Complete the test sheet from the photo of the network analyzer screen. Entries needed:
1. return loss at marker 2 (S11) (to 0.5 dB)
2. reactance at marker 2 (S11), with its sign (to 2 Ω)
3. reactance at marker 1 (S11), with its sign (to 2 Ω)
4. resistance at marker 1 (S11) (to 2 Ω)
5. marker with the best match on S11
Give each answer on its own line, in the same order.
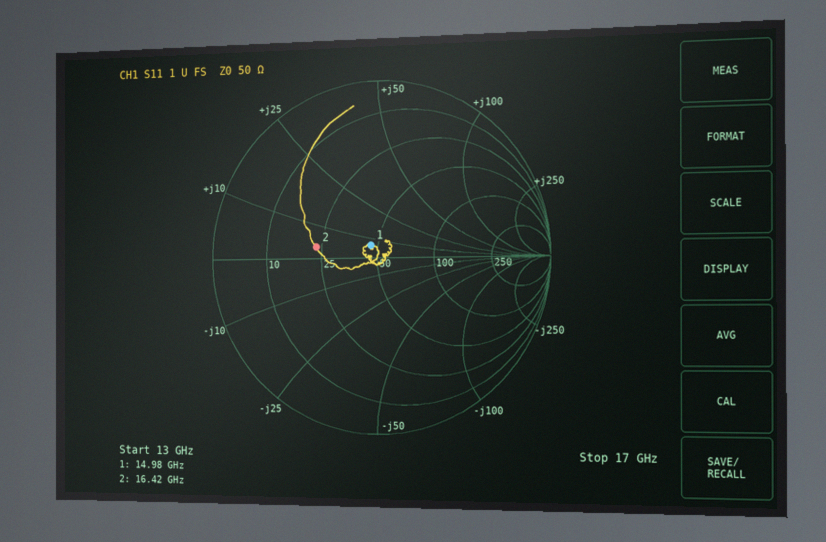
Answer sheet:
8.5 dB
+4 Ω
+6 Ω
46 Ω
marker 1
